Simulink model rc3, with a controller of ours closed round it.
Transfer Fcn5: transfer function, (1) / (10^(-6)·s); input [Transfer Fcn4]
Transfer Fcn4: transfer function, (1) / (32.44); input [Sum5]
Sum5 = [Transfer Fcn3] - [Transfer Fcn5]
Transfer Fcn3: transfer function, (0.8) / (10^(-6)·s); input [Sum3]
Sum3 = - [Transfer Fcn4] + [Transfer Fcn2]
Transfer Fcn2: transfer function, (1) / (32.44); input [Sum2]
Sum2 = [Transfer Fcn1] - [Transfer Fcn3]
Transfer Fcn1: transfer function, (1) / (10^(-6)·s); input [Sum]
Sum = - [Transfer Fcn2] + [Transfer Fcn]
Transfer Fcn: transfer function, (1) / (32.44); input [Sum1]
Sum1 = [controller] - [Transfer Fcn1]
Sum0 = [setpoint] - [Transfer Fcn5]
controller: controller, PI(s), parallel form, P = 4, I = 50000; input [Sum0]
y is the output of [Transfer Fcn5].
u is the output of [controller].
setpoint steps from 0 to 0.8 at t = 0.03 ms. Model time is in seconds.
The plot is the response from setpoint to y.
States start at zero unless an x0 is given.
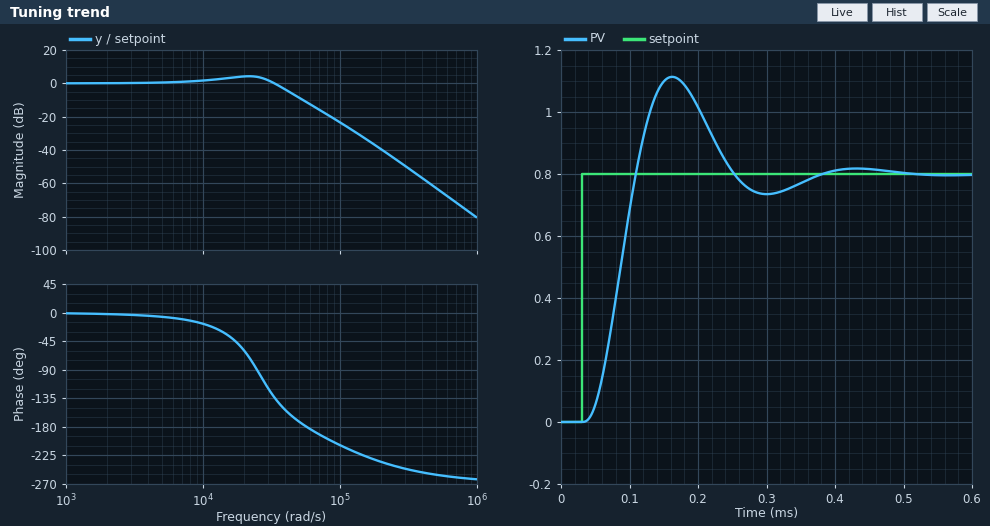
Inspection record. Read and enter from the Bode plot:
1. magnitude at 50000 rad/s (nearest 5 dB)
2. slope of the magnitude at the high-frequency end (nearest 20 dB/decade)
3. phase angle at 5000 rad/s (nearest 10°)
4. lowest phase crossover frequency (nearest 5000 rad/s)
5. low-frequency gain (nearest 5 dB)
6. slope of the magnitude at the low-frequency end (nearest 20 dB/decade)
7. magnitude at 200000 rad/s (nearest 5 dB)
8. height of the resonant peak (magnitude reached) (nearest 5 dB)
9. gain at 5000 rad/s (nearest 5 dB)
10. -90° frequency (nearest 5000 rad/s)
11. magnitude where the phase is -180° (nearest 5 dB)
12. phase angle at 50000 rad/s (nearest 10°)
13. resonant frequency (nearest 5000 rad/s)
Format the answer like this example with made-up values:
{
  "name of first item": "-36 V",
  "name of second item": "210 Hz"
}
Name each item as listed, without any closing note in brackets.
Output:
{
  "magnitude at 50000 rad/s": "-10 dB",
  "slope of the magnitude at the high-frequency end": "-60 dB/decade",
  "phase angle at 5000 rad/s": "-10°",
  "lowest phase crossover frequency": "55000 rad/s",
  "low-frequency gain": "0 dB",
  "slope of the magnitude at the low-frequency end": "0 dB/decade",
  "magnitude at 200000 rad/s": "-40 dB",
  "height of the resonant peak (magnitude reached)": "5 dB",
  "gain at 5000 rad/s": "0 dB",
  "-90° frequency": "25000 rad/s",
  "magnitude where the phase is -180°": "-10 dB",
  "phase angle at 50000 rad/s": "-170°",
  "resonant frequency": "20000 rad/s"
}
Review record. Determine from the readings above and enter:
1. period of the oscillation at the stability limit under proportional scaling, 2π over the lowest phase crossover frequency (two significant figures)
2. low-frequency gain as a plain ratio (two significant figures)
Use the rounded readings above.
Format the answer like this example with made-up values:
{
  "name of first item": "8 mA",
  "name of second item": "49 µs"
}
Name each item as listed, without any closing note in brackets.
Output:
{
  "period of the oscillation at the stability limit under proportional scaling, 2π over the lowest phase crossover frequency": "0.00011 s",
  "low-frequency gain as a plain ratio": "1.0"
}
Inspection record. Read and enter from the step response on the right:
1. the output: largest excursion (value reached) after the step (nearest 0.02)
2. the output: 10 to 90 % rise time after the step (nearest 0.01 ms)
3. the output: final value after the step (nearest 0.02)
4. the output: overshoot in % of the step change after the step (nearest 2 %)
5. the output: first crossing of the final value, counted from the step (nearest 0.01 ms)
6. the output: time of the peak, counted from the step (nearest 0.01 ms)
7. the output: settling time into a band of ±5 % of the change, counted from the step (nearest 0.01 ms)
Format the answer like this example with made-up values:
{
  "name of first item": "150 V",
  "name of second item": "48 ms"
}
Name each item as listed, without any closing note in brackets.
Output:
{
  "the output: largest excursion (value reached) after the step": "1.12",
  "the output: 10 to 90 % rise time after the step": "0.05 ms",
  "the output: final value after the step": "0.80",
  "the output: overshoot in % of the step change after the step": "40 %",
  "the output: first crossing of the final value, counted from the step": "0.08 ms",
  "the output: time of the peak, counted from the step": "0.13 ms",
  "the output: settling time into a band of ±5 % of the change, counted from the step": "0.31 ms"
}
